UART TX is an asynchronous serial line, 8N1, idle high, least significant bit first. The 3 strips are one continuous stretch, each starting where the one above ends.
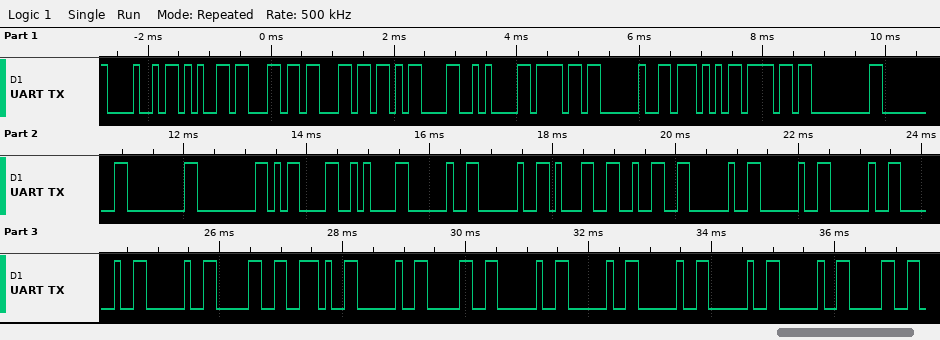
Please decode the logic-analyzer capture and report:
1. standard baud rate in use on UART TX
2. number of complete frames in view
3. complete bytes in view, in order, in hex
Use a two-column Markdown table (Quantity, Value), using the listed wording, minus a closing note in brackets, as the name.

| Quantity | Value |
|---|---|
| standard baud rate in use on UART TX | 9600 baud |
| number of complete frames in view | 35 |
| complete bytes in view, in order, in hex | 48 65 6C 6C 0D 0A 6F 20 57 6F 00 00 00 00 0D 0A 20 20 31 32 20 20 20 20 20 30 2E 20 30 20 20 20 20 20 30 |
